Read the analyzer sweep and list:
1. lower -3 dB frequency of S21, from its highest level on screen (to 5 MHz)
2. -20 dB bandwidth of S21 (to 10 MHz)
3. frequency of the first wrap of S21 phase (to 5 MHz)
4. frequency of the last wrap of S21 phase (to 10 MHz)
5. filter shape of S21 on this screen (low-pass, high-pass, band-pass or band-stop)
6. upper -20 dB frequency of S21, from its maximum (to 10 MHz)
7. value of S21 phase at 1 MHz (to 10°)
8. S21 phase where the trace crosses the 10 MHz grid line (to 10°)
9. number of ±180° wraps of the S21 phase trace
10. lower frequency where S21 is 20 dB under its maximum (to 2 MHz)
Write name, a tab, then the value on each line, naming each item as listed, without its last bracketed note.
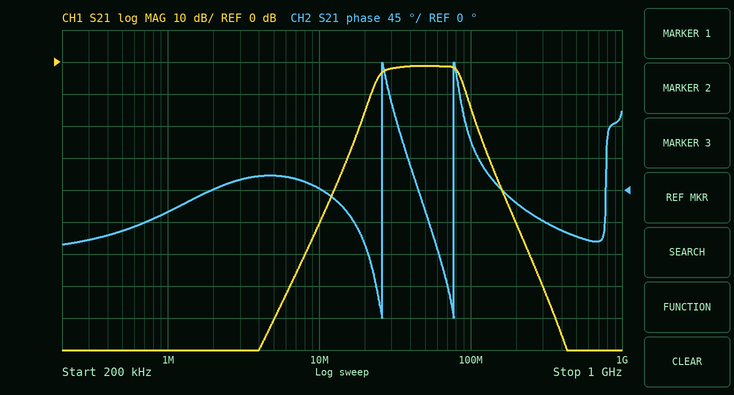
lower -3 dB frequency of S21, from its highest level on screen	25 MHz
-20 dB bandwidth of S21	90 MHz
frequency of the first wrap of S21 phase	25 MHz
frequency of the last wrap of S21 phase	80 MHz
filter shape of S21 on this screen	band-pass
upper -20 dB frequency of S21, from its maximum	110 MHz
value of S21 phase at 1 MHz	-30°
S21 phase where the trace crosses the 10 MHz grid line	0°
number of ±180° wraps of the S21 phase trace	2
lower frequency where S21 is 20 dB under its maximum	18 MHz
